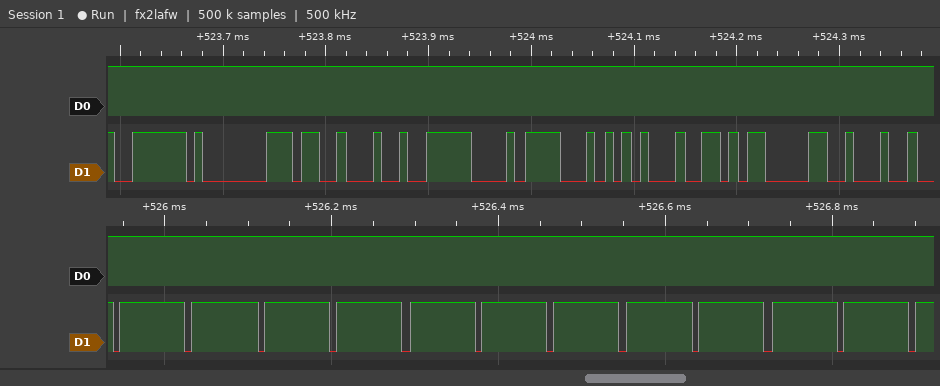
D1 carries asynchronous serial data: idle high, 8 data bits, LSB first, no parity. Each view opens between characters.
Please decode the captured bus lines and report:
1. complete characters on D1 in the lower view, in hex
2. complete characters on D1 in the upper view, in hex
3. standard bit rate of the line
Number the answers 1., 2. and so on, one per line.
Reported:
1. FF, FF, FF, FF, FF, FF, FF, FF, FF, FF, FF
2. 7E, C0, 13, F2, E8, 54, 64, 83, 22
3. 115200 baud
